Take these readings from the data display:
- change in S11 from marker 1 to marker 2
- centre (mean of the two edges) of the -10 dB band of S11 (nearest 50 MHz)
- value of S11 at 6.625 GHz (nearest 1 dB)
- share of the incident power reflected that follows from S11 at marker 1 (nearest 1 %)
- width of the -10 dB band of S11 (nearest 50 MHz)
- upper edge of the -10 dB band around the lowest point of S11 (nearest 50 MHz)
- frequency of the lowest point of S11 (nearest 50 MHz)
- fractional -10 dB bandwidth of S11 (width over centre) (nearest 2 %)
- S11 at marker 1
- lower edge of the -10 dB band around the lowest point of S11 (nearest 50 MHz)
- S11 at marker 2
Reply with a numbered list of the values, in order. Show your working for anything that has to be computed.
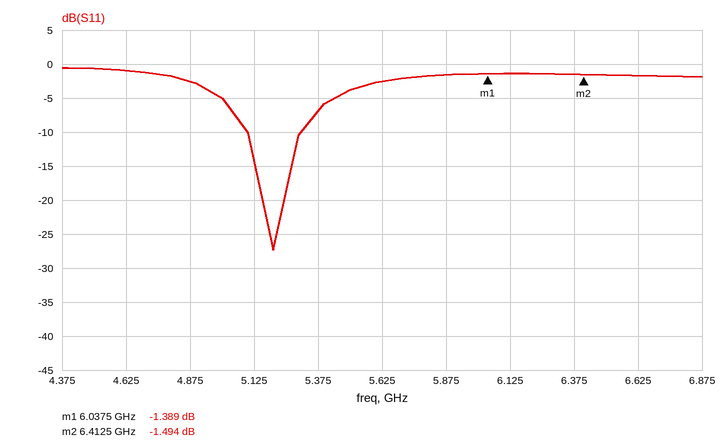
1. -1.494 − (-1.389) = -0.105 dB
2. 5.20 GHz
3. -2 dB
4. 10^(-1.389/10) ≈ 73 %
5. 5.30 GHz − 5.10 GHz = 200 MHz
6. 5.30 GHz
7. 5.20 GHz
8. 200 MHz / 5.2 GHz ≈ 4 %
9. -1.389 dB
10. 5.10 GHz
11. -1.494 dB
